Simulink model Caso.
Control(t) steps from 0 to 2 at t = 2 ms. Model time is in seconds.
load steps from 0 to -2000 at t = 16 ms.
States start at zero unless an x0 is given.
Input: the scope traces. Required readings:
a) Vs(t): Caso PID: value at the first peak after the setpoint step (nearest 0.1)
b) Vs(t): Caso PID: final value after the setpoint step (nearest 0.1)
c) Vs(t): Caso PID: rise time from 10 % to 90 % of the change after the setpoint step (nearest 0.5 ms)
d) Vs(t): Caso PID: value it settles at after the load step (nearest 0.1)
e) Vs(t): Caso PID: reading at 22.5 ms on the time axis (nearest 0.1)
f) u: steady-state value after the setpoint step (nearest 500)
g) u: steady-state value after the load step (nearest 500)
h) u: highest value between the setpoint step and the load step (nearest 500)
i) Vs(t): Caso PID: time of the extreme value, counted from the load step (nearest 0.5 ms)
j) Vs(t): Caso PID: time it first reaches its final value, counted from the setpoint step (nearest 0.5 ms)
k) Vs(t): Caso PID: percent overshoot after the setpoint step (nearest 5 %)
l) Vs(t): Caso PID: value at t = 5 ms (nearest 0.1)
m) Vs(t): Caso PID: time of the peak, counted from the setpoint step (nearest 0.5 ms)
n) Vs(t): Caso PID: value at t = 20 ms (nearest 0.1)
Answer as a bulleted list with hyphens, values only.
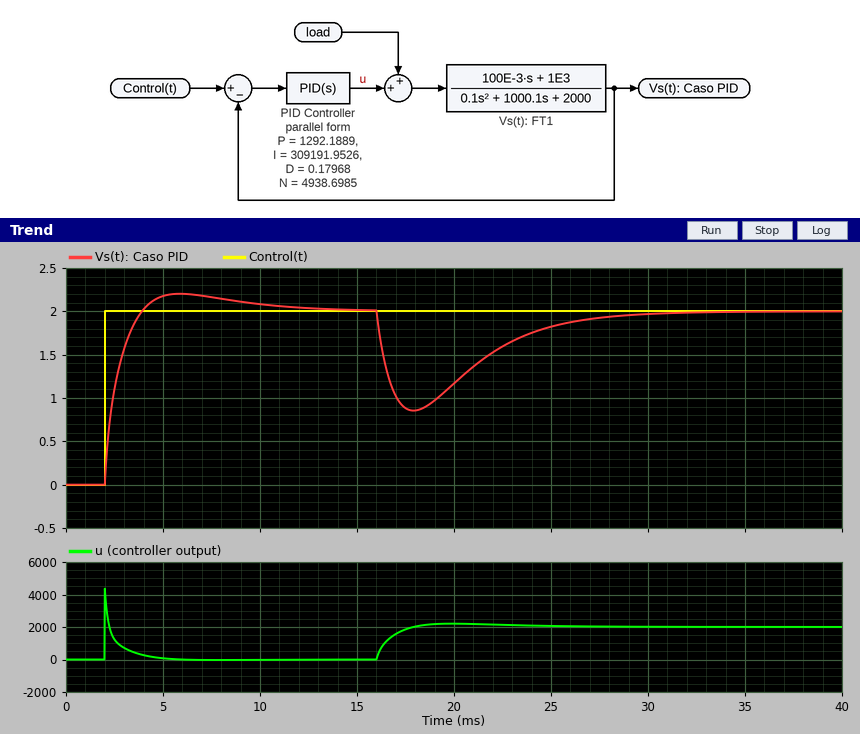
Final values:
- 2.2
- 2.0
- 1.5 ms
- 2.0
- 1.6
- 0
- 2000
- 4500
- 2.0 ms
- 2.0 ms
- 10 %
- 2.2
- 4.0 ms
- 1.2
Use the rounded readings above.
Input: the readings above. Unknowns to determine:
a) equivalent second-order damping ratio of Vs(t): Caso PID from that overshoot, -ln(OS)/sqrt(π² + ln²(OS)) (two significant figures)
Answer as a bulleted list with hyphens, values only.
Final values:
- 0.59
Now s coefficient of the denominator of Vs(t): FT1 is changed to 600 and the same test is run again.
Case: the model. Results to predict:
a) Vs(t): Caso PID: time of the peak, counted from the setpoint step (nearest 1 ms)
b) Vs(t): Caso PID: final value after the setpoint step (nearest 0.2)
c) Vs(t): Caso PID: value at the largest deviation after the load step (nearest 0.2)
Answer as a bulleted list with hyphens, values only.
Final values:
- 3 ms
- 2.0
- 0.8
